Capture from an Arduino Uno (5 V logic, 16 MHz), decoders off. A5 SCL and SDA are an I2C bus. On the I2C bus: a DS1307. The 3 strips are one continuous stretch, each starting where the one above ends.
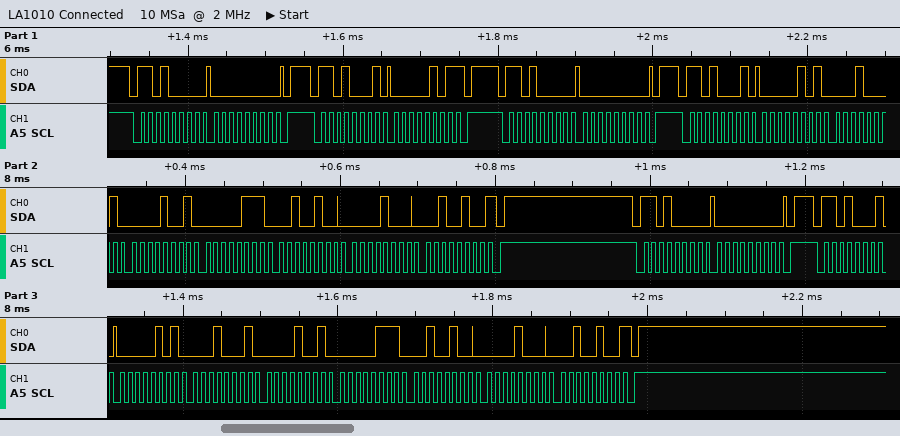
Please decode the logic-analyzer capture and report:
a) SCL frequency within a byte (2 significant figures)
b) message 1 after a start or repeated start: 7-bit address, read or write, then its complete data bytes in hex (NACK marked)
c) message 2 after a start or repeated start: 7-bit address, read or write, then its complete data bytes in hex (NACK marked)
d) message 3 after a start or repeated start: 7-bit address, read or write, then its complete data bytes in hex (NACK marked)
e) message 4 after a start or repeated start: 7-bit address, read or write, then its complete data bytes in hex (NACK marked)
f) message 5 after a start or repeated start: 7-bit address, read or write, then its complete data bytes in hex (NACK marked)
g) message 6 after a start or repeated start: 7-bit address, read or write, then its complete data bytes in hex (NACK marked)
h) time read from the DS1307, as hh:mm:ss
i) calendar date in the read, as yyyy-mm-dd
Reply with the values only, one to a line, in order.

100 kHz
0x68 write: 00
0x68 read: 05 NACK
0x68 write: 00
0x68 read: 05 11 09 07 24 08 24 NACK
0x68 write: 00
0x68 read: 05 11 09 07 24 08 24 NACK
09:11:05
2024-08-24
